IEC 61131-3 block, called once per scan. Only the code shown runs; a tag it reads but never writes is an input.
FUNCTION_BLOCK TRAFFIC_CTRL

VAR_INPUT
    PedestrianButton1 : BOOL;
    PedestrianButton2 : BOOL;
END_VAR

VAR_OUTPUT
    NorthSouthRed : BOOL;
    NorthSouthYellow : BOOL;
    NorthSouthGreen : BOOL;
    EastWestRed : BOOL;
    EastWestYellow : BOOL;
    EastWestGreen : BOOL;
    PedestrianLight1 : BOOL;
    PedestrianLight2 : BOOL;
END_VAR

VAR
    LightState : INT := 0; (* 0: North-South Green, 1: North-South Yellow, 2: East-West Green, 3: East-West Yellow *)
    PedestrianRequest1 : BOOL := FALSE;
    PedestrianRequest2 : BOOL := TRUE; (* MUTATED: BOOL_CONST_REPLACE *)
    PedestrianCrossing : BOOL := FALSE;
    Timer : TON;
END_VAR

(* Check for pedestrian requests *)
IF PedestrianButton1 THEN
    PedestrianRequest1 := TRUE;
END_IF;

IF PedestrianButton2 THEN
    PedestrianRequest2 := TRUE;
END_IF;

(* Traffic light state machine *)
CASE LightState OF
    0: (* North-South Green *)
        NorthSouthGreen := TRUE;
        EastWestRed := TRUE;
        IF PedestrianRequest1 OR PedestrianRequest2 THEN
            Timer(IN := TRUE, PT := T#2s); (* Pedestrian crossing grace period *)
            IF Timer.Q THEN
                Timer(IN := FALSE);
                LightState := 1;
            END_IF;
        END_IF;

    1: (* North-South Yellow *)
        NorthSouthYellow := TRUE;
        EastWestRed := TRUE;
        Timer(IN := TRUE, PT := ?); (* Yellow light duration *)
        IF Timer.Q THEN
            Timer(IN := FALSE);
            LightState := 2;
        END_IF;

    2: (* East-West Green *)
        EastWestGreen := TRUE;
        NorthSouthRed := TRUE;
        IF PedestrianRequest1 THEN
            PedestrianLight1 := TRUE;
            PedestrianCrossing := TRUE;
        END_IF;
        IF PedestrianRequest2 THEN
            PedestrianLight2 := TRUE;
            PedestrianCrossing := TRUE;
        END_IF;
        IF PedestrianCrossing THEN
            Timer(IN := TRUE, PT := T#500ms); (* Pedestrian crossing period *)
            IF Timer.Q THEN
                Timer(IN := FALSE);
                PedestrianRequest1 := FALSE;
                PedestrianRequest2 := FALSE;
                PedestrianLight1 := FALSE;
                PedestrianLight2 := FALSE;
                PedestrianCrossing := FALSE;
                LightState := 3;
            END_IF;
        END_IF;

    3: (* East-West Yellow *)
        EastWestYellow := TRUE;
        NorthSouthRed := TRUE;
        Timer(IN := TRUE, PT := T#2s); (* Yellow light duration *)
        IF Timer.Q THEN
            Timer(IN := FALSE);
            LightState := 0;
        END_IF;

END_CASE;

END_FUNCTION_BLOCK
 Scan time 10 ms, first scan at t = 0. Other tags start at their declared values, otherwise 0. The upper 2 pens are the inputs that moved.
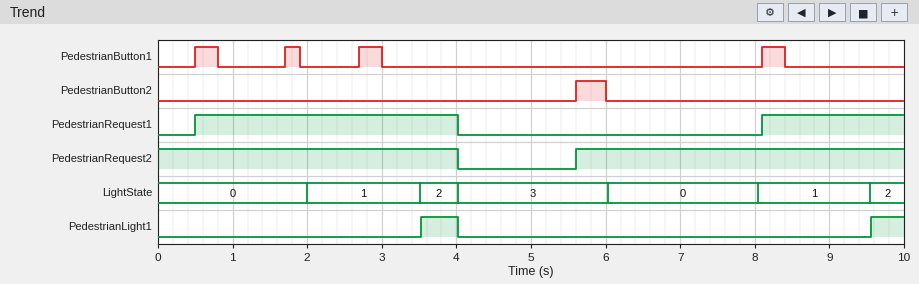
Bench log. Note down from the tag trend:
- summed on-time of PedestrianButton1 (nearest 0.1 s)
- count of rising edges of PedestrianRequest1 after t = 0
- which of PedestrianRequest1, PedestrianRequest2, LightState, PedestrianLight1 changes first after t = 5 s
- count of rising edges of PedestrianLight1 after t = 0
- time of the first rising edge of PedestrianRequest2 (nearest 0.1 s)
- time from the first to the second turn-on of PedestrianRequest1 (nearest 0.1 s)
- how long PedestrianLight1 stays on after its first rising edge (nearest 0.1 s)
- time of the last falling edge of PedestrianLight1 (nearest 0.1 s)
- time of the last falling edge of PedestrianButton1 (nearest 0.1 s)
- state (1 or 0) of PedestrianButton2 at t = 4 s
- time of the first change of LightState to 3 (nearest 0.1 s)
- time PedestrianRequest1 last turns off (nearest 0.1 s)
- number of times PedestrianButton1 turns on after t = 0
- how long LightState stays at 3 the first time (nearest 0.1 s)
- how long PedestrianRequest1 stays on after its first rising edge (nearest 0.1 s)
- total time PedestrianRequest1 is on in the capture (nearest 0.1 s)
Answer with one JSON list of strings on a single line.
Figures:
["1.1 s", "2", "PedestrianRequest2", "2", "5.6 s", "7.6 s", "0.5 s", "4.0 s", "8.4 s", "0", "4.0 s", "4.0 s", "4", "2.0 s", "3.5 s", "5.4 s"]
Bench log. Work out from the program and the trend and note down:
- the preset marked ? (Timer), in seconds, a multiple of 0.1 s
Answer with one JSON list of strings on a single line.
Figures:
["1.5 s"]
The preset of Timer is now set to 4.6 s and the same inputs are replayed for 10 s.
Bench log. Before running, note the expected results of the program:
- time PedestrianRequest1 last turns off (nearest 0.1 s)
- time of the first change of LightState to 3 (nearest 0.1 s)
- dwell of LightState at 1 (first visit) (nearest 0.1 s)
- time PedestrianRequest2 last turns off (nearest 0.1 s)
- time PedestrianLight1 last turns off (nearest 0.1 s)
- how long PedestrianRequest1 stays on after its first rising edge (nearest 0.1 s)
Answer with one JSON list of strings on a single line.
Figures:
["7.1 s", "7.1 s", "4.6 s", "7.1 s", "7.1 s", "6.6 s"]
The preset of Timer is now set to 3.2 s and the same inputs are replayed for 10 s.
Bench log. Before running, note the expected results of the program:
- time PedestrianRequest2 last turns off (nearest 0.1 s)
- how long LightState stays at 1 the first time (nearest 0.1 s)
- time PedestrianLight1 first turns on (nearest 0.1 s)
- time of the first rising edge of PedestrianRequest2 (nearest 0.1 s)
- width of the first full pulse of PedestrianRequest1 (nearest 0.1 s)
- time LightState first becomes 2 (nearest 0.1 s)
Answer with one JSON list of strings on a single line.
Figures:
["5.7 s", "3.2 s", "5.2 s", "5.7 s", "5.2 s", "5.2 s"]
